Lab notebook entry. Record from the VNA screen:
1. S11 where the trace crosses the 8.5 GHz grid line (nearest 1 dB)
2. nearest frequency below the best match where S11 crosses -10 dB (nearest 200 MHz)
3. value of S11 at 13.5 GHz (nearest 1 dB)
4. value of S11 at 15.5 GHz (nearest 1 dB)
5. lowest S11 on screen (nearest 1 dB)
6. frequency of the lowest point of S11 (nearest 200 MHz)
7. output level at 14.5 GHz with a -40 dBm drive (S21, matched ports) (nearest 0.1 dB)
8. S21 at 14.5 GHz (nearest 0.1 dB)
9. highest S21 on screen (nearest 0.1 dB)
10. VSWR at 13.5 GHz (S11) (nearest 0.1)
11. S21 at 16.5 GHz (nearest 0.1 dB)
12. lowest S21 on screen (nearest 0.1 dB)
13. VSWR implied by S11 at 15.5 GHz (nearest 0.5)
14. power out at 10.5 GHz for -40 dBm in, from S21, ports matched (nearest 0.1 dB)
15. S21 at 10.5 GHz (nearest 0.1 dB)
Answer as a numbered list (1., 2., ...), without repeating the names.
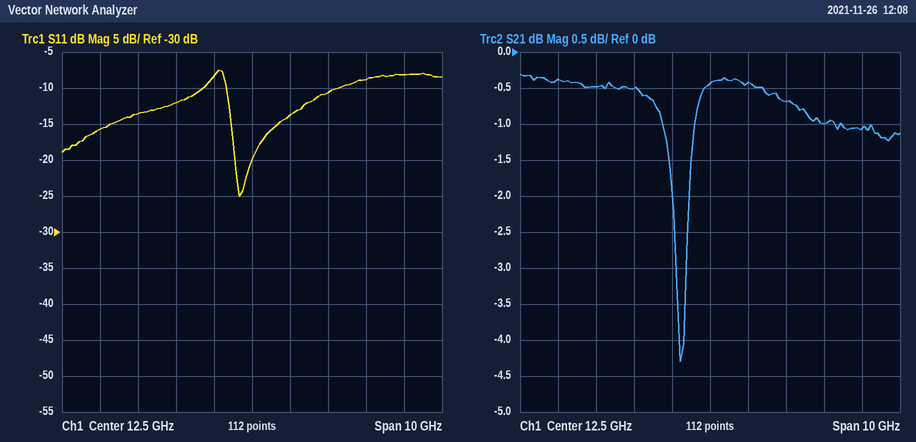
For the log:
1. -16 dB
2. 11.8 GHz
3. -14 dB
4. -9 dB
5. -25 dB
6. 12.2 GHz
7. -40.7 dBm
8. -0.7 dB
9. -0.3 dB
10. 1.5
11. -1.1 dB
12. -4.3 dB
13. 2.0
14. -40.5 dBm
15. -0.5 dB
